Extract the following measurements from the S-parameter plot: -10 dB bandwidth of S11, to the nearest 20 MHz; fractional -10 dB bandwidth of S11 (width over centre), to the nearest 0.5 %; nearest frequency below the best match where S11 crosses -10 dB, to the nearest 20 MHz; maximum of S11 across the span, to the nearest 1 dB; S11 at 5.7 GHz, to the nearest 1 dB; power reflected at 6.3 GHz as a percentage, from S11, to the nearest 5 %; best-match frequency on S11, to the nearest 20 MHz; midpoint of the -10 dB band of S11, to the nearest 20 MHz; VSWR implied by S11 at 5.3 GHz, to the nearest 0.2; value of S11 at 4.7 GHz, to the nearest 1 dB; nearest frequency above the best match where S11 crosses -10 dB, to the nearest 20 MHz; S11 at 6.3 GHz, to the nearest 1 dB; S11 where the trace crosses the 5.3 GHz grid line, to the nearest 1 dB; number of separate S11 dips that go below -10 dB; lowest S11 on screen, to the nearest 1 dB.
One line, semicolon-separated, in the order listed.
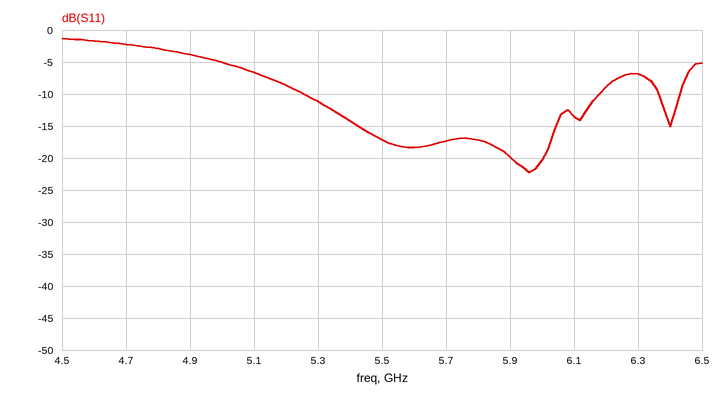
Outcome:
920 MHz; 16.0 %; 5.26 GHz; -1 dB; -17 dB; 20 %; 5.96 GHz; 5.72 GHz; 1.8; -2 dB; 6.18 GHz; -7 dB; -11 dB; 2; -22 dB
